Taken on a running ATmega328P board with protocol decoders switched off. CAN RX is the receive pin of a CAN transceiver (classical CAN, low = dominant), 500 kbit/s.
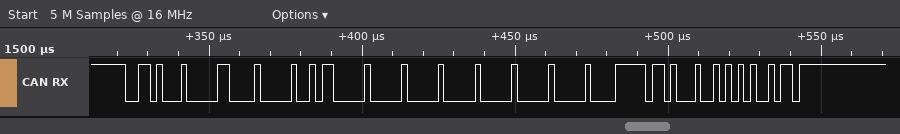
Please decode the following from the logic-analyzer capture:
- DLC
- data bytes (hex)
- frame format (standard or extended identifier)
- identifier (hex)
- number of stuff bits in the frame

8
40 58 00 00 00 00 0F E8
standard
0x344
10
